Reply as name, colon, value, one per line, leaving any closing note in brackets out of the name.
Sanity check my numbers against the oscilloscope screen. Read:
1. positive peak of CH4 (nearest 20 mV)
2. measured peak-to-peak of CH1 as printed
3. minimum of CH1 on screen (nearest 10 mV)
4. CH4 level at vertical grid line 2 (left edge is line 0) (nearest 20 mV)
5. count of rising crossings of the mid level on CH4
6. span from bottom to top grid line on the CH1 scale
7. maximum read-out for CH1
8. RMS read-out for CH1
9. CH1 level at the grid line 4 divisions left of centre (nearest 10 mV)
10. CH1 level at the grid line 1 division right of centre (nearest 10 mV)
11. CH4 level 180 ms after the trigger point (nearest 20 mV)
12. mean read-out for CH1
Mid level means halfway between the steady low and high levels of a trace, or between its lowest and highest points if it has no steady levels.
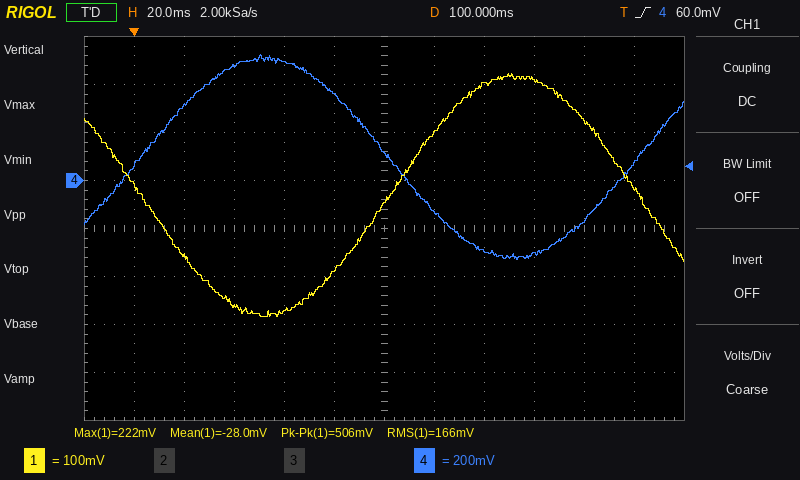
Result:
positive peak of CH4: 520 mV
measured peak-to-peak of CH1 as printed: 506 mV
minimum of CH1 on screen: -280 mV
CH4 level at vertical grid line 2 (left edge is line 0): 320 mV
count of rising crossings of the mid level on CH4: 2
span from bottom to top grid line on the CH1 scale: 800 mV
maximum read-out for CH1: 222 mV
RMS read-out for CH1: 166 mV
CH1 level at the grid line 4 divisions left of centre: -160 mV
CH1 level at the grid line 1 division right of centre: 100 mV
CH4 level 180 ms after the trigger point: -160 mV
mean read-out for CH1: -28.0 mV
